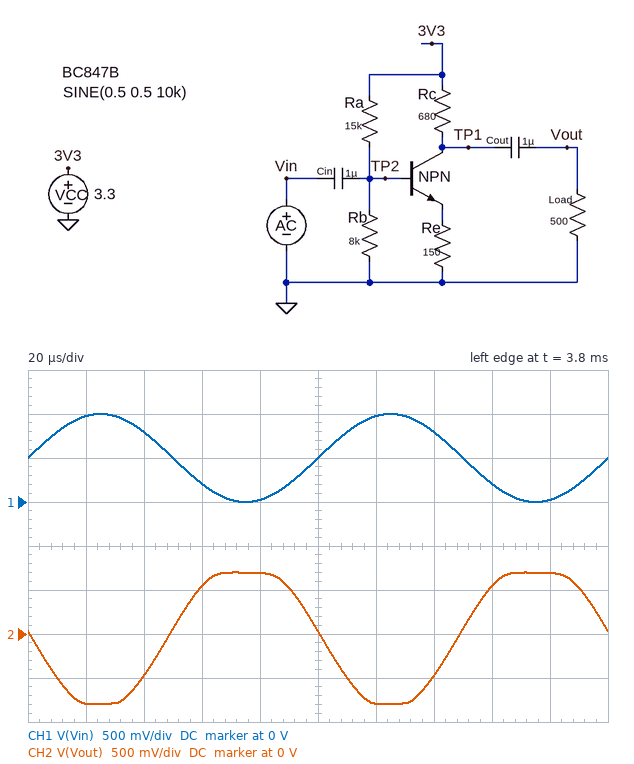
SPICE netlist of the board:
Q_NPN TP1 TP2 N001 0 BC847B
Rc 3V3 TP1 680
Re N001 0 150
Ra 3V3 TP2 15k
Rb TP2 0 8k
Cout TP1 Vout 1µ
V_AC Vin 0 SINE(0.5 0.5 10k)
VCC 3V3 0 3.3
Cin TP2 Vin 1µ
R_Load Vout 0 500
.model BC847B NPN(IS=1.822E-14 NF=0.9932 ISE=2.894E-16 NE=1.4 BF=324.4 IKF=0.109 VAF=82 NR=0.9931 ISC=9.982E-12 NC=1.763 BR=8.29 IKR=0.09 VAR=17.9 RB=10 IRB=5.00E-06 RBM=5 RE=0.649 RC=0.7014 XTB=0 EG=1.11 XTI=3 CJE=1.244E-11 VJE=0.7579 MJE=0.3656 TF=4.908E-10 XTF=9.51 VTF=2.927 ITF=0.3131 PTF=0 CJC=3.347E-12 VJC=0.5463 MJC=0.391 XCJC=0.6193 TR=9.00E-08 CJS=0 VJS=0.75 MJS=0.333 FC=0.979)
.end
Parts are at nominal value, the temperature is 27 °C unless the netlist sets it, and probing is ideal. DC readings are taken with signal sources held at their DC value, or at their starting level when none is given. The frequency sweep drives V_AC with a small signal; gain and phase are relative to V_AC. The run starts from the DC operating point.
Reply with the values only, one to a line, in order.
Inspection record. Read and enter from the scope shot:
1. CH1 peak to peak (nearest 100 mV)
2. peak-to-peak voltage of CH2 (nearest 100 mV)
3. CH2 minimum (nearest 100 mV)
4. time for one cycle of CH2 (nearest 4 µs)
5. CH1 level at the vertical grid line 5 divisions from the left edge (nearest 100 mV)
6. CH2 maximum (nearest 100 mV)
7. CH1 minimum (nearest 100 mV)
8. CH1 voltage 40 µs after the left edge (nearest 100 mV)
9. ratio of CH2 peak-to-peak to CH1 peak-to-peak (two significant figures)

1.0 V
1.5 V
-800 mV
100 µs
500 mV
700 mV
0 V
800 mV
1.5
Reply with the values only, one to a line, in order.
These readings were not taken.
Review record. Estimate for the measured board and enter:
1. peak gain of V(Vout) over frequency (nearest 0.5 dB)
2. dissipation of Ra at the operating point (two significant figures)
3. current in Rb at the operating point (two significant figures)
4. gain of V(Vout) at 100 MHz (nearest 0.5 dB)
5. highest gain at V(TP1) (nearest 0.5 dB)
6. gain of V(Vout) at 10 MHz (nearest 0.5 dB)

5.0 dB
320 µW
140 µA
4.5 dB
11.0 dB
5.0 dB
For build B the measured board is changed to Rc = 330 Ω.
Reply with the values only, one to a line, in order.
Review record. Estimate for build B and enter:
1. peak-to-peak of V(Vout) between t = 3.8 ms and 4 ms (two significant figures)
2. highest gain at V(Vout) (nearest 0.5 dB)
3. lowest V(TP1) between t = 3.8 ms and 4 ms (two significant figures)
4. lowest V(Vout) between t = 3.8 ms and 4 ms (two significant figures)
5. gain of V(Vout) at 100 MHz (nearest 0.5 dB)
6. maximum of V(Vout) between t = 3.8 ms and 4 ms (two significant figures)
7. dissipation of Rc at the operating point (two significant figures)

1.2 V
2.0 dB
1.7 V
-610 mV
1.5 dB
560 mV
2.7 mW
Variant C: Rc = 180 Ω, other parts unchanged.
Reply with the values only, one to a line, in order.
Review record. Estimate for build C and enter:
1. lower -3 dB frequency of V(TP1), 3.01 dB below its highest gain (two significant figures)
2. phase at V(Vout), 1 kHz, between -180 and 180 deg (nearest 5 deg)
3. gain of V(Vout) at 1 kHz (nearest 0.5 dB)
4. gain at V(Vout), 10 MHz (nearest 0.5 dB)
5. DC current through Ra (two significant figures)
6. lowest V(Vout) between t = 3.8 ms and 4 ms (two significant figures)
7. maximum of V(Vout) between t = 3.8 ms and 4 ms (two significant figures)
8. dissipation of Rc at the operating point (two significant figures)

29 Hz
-165 deg
-2.0 dB
-1.5 dB
150 µA
-410 mV
380 mV
1.5 mW
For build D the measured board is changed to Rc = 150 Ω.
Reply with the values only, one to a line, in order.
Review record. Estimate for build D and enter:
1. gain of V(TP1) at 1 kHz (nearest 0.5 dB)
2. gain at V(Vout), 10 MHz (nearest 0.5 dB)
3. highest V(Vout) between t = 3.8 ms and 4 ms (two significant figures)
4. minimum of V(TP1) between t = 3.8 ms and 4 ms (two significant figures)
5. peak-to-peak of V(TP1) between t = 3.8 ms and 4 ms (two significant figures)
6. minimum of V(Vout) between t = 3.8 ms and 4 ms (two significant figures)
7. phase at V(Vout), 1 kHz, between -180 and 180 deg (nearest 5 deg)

-2.5 dB
-3.0 dB
330 mV
2.5 V
680 mV
-360 mV
-165 deg
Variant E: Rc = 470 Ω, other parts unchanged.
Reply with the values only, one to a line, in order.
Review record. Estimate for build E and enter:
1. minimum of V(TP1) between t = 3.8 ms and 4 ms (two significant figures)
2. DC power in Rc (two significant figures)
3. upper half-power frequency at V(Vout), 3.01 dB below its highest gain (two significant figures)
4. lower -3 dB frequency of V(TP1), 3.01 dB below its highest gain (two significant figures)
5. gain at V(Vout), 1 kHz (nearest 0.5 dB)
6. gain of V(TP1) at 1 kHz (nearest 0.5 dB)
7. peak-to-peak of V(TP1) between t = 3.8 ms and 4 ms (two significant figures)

1.2 V
3.9 mW
620 MHz
26 Hz
3.5 dB
4.0 dB
1.4 V
